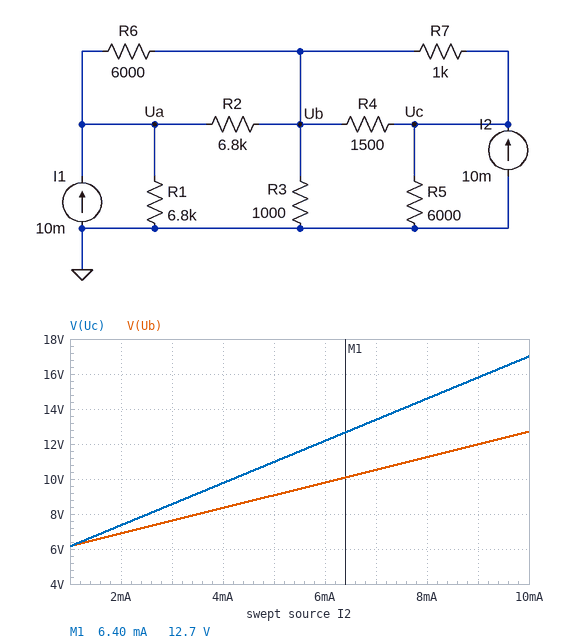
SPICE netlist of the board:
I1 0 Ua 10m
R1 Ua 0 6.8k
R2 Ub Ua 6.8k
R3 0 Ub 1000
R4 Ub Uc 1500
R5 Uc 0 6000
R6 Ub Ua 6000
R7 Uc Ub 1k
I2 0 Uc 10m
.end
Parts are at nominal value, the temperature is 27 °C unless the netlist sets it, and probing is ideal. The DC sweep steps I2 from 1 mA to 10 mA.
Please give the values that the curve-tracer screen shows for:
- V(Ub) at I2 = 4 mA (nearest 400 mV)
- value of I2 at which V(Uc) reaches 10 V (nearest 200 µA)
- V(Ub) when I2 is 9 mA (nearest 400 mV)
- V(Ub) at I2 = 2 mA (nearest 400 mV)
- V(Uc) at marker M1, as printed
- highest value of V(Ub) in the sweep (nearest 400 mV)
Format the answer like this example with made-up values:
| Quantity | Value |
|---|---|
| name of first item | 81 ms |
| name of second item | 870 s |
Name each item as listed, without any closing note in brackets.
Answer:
| Quantity | Value |
|---|---|
| V(Ub) at I2 = 4 mA | 8.4 V |
| value of I2 at which V(Uc) reaches 10 V | 4.2 mA |
| V(Ub) when I2 is 9 mA | 12.0 V |
| V(Ub) at I2 = 2 mA | 6.8 V |
| V(Uc) at marker M1, as printed | 12.7 V |
| highest value of V(Ub) in the sweep | 12.8 V |
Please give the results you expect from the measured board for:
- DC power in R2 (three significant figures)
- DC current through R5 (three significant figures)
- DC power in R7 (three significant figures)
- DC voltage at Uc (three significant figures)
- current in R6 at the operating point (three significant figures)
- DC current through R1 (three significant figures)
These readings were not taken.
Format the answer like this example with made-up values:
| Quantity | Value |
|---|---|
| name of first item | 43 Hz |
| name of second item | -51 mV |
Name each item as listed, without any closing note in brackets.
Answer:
| Quantity | Value |
|---|---|
| DC power in R2 | 45.8 mW |
| DC current through R5 | 2.83 mA |
| DC power in R7 | 18.5 mW |
| DC voltage at Uc | 17.0 V |
| current in R6 at the operating point | 2.94 mA |
| DC current through R1 | 4.46 mA |
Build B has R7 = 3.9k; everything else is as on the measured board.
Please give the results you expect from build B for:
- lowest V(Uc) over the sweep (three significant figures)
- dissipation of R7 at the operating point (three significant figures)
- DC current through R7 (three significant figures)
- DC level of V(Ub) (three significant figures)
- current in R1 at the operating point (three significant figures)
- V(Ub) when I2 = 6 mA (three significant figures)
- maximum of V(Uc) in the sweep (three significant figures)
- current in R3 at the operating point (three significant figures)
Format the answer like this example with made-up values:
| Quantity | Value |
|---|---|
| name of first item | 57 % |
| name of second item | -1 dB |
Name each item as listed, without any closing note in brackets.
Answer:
| Quantity | Value |
|---|---|
| lowest V(Uc) over the sweep | 6.14 V |
| dissipation of R7 at the operating point | 13.6 mW |
| DC current through R7 | 1.87 mA |
| DC level of V(Ub) | 12.3 V |
| current in R1 at the operating point | 4.42 mA |
| V(Ub) when I2 = 6 mA | 9.58 V |
| maximum of V(Uc) in the sweep | 19.6 V |
| current in R3 at the operating point | 12.3 mA |
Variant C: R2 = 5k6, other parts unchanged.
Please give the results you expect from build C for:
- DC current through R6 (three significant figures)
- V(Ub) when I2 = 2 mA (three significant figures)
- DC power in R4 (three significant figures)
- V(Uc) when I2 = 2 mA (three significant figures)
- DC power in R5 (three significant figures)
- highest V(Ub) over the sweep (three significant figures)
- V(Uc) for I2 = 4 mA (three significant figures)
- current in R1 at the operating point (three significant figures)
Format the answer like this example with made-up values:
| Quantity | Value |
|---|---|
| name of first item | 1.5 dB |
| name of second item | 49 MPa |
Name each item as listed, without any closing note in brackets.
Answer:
| Quantity | Value |
|---|---|
| DC current through R6 | 2.75 mA |
| V(Ub) when I2 = 2 mA | 7.04 V |
| DC power in R4 | 12.3 mW |
| V(Uc) when I2 = 2 mA | 7.49 V |
| DC power in R5 | 48.9 mW |
| highest V(Ub) over the sweep | 12.8 V |
| V(Uc) for I2 = 4 mA | 9.90 V |
| current in R1 at the operating point | 4.31 mA |
